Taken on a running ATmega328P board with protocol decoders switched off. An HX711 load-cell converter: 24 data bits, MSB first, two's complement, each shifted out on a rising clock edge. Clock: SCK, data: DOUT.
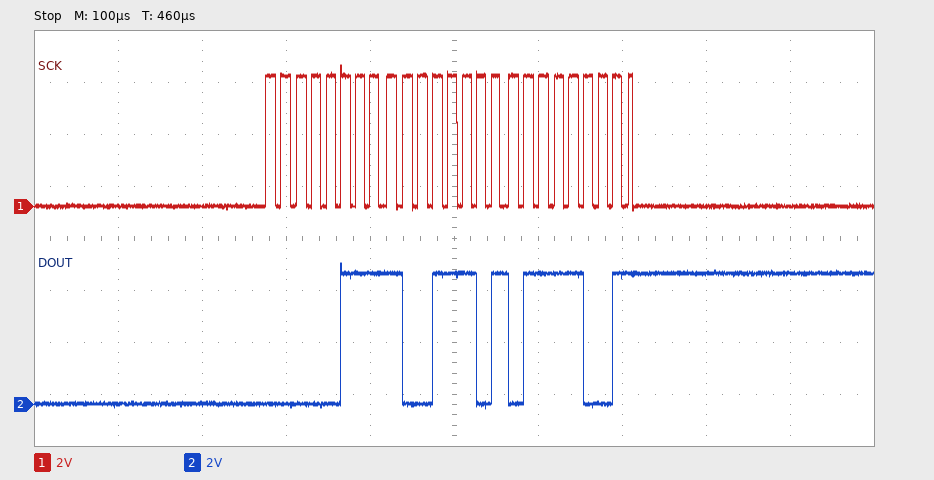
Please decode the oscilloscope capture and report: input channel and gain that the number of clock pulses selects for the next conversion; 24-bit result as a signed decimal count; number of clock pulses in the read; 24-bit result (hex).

channel A, gain 128
499065
25
0x079D79
